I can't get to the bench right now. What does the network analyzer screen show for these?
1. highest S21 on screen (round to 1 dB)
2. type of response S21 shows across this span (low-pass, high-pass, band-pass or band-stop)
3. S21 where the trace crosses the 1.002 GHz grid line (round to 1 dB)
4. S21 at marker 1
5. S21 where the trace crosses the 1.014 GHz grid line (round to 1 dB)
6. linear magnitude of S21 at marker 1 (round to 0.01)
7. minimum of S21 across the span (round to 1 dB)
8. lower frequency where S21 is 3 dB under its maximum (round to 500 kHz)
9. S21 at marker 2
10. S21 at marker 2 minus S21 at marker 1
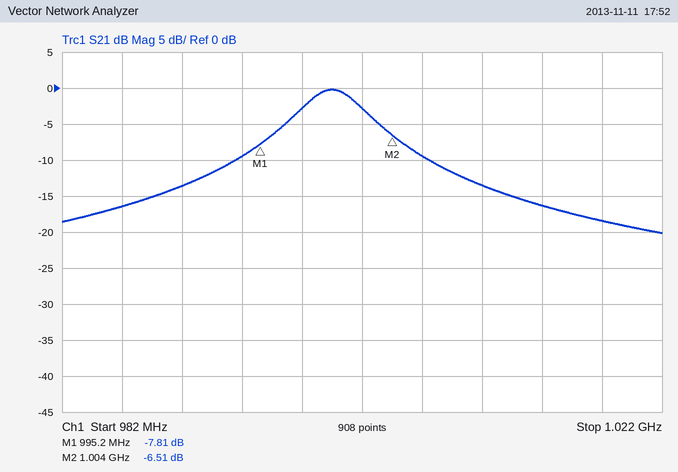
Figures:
0 dB
band-pass
-3 dB
-7.81 dB
-16 dB
0.41
-20 dB
998.0 MHz
-6.51 dB
1.30 dB
